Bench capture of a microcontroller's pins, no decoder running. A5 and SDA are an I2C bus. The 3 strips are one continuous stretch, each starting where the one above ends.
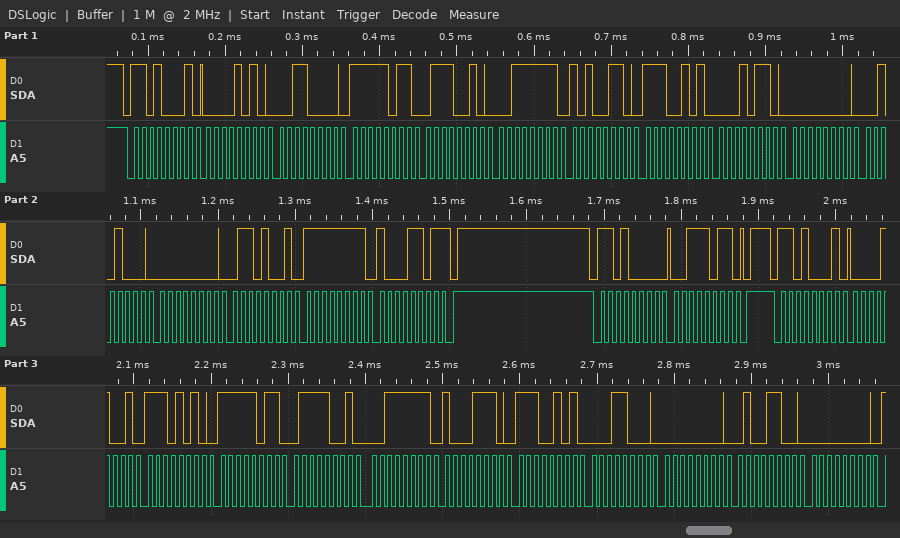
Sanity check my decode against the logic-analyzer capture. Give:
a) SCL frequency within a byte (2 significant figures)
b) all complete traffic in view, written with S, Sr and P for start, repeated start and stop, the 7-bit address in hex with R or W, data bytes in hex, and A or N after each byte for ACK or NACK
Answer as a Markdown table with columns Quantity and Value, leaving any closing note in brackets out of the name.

| Quantity | Value |
|---|---|
| SCL frequency within a byte | 100 kHz |
| all complete traffic in view, written with S, Sr and P for start, repeated start and stop, the 7-bit address in hex with R or W, data bytes in hex, and A or N after each byte for ACK or NACK | S 68R A 0A A 30 A FB A 72 A 3F A A6 A E5 A 16 A 00 A 28 A 00 A 69 A FF A 8D N P S 68W A 3B A P S 68R A 09 A EA A FB A 79 A 3F A 8E A E5 A 18 A 00 A 4C A 00 A |
